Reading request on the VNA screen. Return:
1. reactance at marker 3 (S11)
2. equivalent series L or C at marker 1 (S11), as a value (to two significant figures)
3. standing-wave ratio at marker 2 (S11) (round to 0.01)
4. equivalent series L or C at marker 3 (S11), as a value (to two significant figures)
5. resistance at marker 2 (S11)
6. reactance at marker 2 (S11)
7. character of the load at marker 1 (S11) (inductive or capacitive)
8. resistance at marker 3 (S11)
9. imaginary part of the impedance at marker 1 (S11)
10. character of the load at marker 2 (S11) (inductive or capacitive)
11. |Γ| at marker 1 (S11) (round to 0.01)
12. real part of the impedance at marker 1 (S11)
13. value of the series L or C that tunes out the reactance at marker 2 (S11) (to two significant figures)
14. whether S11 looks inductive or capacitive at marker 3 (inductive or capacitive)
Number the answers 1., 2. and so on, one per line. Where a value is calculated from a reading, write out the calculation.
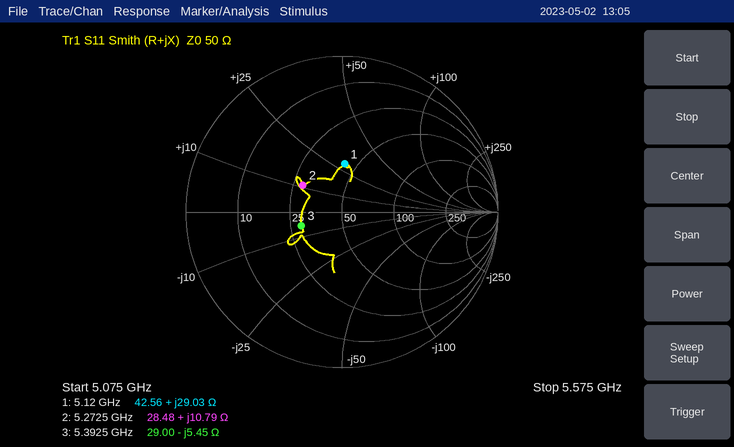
1. -5.45 Ω
2. L = 29.03 Ω/(2π × 5.12 GHz) ≈ 902 pH, so 900 pH to two significant figures
3. 1.87
4. C = 1/(2π × 5.3925 GHz × 5.45 Ω) ≈ 5.4 pF
5. 28.48 Ω
6. +10.79 Ω
7. inductive
8. 29.00 Ω
9. +29.03 Ω
10. inductive
11. 0.31
12. 42.56 Ω
13. C = 1/(2π × 5.2725 GHz × 10.79 Ω) ≈ 2.8 pF
14. capacitive
